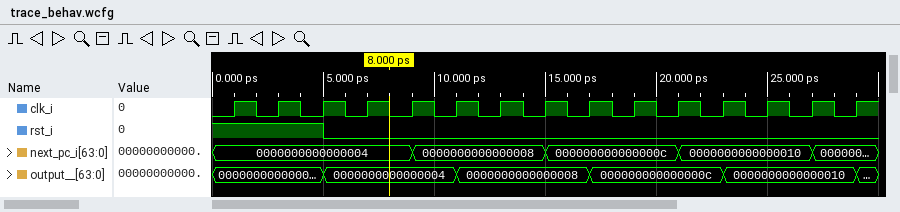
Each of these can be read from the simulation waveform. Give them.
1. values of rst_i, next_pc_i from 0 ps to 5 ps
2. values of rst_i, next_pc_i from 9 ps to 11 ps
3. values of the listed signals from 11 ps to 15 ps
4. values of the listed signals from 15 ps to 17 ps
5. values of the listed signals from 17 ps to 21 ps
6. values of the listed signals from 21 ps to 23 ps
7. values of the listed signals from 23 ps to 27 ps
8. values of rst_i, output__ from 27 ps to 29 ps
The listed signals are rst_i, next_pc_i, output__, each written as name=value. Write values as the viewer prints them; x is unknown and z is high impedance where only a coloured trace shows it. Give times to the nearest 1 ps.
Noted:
rst_i=1, next_pc_i=0000000000000004
rst_i=0, next_pc_i=0000000000000008
rst_i=0, next_pc_i=0000000000000008, output__=0000000000000008
rst_i=0, next_pc_i=000000000000000c, output__=0000000000000008
rst_i=0, next_pc_i=000000000000000c, output__=000000000000000c
rst_i=0, next_pc_i=0000000000000010, output__=000000000000000c
rst_i=0, next_pc_i=0000000000000010, output__=0000000000000010
rst_i=0, output__=0000000000000010
